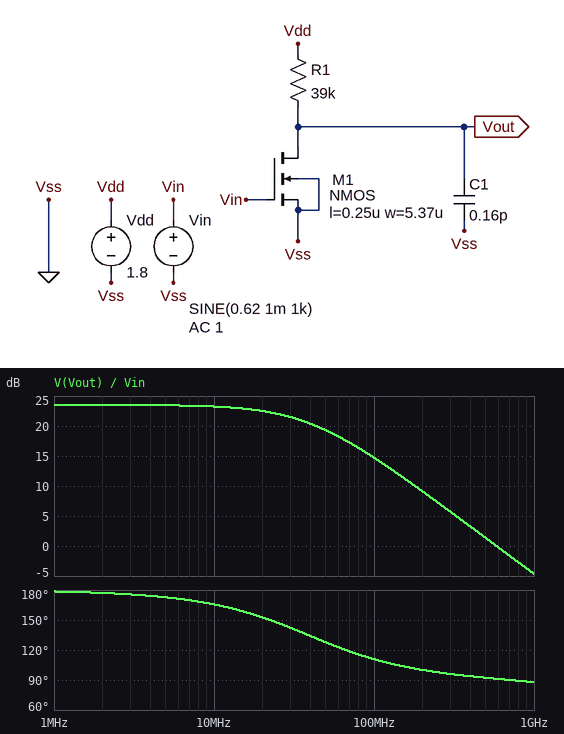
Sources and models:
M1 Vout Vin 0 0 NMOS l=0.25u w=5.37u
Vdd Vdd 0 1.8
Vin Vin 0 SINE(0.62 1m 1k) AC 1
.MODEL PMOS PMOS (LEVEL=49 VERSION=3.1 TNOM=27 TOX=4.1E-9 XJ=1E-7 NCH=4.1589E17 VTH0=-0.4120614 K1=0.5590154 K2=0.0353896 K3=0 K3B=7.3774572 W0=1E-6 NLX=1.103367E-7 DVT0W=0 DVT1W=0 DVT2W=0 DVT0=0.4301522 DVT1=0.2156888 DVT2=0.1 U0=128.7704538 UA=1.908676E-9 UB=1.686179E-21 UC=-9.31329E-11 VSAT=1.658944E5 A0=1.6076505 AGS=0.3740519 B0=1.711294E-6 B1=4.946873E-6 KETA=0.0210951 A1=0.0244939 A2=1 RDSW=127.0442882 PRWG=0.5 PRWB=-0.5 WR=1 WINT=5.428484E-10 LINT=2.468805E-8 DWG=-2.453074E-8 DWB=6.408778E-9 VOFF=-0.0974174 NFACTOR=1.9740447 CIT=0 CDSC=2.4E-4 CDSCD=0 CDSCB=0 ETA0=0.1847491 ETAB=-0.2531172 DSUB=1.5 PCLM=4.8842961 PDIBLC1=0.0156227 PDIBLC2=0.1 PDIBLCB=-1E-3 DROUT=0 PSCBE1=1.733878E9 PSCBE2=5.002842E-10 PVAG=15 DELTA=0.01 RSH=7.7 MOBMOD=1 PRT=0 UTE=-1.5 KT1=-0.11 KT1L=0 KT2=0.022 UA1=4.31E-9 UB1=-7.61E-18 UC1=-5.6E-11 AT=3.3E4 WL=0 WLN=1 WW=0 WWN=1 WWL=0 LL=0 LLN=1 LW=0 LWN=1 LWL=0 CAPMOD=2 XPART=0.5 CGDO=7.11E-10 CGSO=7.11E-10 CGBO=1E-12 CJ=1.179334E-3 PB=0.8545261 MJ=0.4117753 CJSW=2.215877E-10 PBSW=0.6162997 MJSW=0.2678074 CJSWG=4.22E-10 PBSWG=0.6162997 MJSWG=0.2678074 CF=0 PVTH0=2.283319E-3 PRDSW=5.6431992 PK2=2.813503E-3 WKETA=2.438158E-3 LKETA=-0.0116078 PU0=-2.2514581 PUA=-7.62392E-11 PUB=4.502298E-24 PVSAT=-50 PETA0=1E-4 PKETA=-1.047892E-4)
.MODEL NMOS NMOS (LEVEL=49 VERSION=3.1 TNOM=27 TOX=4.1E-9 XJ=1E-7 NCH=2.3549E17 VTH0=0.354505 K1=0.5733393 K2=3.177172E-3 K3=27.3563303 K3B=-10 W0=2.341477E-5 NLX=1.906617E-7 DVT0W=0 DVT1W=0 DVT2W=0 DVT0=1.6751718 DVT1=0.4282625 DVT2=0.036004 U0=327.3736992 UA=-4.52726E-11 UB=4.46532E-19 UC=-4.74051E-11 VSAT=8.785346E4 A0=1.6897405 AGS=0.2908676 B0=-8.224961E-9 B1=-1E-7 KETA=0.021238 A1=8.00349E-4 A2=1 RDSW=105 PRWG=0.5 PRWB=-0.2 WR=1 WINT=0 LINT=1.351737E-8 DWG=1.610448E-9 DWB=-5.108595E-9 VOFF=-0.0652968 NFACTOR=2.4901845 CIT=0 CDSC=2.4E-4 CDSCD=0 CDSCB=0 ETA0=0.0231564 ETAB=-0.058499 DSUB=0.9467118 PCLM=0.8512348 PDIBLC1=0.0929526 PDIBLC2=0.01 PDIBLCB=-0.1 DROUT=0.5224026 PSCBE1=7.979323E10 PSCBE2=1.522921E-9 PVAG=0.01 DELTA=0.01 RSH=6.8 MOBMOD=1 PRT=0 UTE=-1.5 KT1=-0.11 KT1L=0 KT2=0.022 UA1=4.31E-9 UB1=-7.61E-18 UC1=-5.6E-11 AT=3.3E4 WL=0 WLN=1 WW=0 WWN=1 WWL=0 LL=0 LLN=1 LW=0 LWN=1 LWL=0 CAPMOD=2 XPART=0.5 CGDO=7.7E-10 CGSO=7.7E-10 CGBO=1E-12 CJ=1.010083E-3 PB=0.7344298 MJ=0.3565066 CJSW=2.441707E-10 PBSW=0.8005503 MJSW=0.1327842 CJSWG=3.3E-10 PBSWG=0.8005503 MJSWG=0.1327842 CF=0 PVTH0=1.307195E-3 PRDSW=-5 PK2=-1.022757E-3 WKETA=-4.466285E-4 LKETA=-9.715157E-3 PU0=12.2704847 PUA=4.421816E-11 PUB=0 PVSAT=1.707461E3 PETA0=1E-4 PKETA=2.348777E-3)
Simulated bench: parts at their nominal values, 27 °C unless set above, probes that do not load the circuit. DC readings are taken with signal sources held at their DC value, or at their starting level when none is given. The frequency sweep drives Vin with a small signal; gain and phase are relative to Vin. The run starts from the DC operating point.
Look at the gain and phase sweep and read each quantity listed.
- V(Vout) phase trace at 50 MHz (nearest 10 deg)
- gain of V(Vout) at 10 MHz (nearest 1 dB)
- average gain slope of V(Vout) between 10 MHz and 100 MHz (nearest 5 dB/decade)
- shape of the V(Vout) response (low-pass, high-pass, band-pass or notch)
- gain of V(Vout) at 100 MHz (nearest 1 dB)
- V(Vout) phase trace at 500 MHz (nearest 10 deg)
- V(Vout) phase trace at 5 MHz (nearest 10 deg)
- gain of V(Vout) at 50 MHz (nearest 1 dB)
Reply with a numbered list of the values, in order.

1. 130 deg
2. 23 dB
3. -10 dB/decade
4. low-pass
5. 15 dB
6. 90 deg
7. 170 deg
8. 19 dB
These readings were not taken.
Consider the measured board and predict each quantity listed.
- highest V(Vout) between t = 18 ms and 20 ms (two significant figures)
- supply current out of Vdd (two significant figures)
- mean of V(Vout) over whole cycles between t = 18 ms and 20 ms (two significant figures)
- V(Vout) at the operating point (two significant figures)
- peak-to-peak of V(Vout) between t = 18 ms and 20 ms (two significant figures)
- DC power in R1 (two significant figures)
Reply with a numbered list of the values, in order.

1. 270 mV
2. 40 µA
3. 260 mV
4. 260 mV
5. 30 mV
6. 61 µW
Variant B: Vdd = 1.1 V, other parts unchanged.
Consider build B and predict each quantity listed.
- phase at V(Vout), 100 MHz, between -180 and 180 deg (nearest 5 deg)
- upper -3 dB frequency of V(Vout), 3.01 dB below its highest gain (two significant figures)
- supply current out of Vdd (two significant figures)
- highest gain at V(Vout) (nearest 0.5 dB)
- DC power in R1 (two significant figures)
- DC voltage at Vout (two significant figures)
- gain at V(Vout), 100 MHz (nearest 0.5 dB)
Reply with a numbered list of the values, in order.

1. 160 deg
2. 280 MHz
3. 27 µA
4. 1.0 dB
5. 28 µW
6. 61 mV
7. 0.5 dB
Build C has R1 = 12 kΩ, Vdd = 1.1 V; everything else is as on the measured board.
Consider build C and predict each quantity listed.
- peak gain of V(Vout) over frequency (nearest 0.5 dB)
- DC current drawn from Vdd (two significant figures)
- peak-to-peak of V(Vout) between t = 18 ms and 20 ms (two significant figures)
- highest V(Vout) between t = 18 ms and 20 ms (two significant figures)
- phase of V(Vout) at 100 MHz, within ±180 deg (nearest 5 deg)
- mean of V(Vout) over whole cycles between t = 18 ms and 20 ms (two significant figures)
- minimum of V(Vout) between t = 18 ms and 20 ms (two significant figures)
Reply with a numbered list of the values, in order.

1. 17.0 dB
2. 43 µA
3. 14 mV
4. 590 mV
5. 130 deg
6. 580 mV
7. 570 mV
